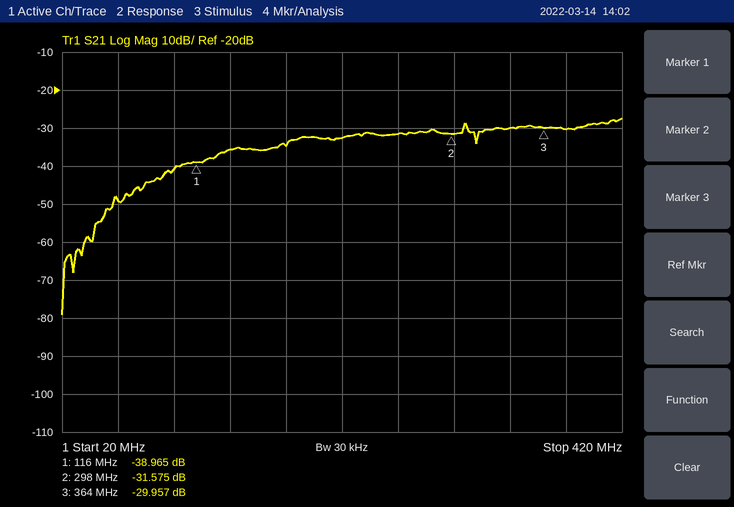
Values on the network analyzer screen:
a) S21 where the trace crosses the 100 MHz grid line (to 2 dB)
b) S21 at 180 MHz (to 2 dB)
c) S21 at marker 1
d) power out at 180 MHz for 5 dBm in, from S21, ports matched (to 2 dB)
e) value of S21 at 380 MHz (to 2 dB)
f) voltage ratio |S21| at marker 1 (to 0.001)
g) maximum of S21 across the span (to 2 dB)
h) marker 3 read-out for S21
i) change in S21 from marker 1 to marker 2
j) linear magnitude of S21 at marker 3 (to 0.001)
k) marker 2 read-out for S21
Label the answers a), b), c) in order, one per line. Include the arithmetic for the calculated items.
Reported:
a) -40 dB
b) -34 dB
c) -38.965 dB
d) 5 dBm + (-34 dB) = -30 dBm
e) -30 dB
f) 10^(-38.965/20) ≈ 0.011
g) -28 dB
h) -29.957 dB
i) -31.575 − (-38.965) = 7.390 dB
j) 10^(-29.957/20) ≈ 0.032
k) -31.575 dB
